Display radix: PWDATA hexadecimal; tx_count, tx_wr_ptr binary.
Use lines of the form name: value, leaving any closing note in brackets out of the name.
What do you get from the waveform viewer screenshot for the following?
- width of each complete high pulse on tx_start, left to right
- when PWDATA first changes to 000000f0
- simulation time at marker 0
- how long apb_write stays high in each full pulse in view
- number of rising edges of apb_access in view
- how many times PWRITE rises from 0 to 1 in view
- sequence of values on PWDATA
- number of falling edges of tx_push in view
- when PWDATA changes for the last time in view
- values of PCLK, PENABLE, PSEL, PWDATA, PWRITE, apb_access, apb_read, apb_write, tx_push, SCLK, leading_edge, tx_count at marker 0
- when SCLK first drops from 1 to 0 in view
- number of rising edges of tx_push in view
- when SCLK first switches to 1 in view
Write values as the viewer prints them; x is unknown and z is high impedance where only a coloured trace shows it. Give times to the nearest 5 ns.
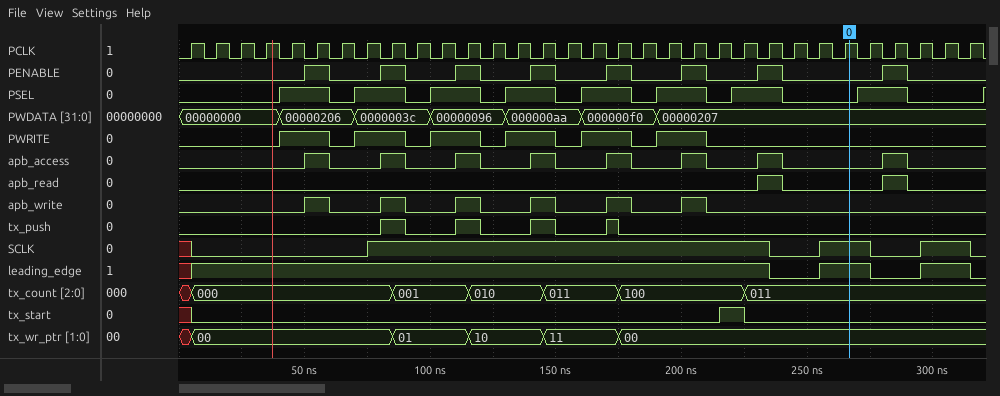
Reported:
width of each complete high pulse on tx_start, left to right: 10 ns
when PWDATA first changes to 000000f0: 160 ns
simulation time at marker 0: 265 ns
how long apb_write stays high in each full pulse in view: 10 ns, 10 ns, 10 ns, 10 ns, 10 ns, 10 ns
number of rising edges of apb_access in view: 8
how many times PWRITE rises from 0 to 1 in view: 6
sequence of values on PWDATA: 00000000, 00000206, 0000003c, 00000096, 000000aa, 000000f0, 00000207
number of falling edges of tx_push in view: 4
when PWDATA changes for the last time in view: 190 ns
values of PCLK, PENABLE, PSEL, PWDATA, PWRITE, apb_access, apb_read, apb_write, tx_push, SCLK, leading_edge, tx_count at marker 0: PCLK=1, PENABLE=0, PSEL=0, PWDATA=00000207, PWRITE=0, apb_access=0, apb_read=0, apb_write=0, tx_push=0, SCLK=1, leading_edge=1, tx_count=011
when SCLK first drops from 1 to 0 in view: 235 ns
number of rising edges of tx_push in view: 4
when SCLK first switches to 1 in view: 75 ns
